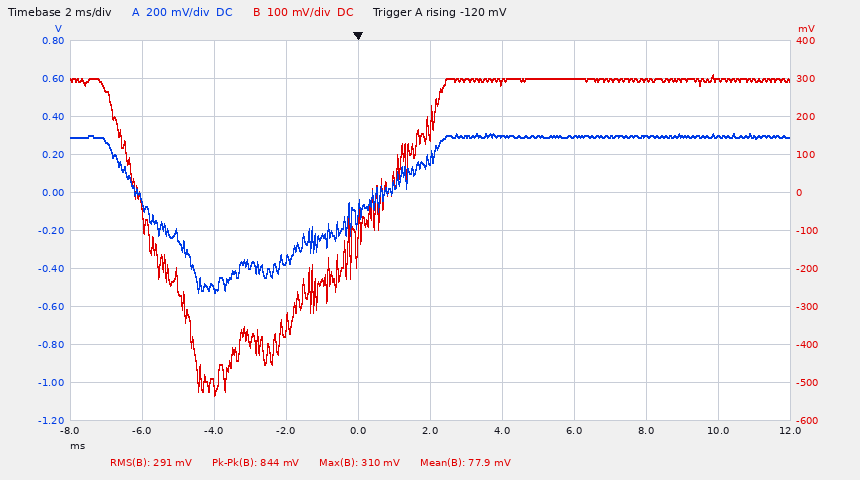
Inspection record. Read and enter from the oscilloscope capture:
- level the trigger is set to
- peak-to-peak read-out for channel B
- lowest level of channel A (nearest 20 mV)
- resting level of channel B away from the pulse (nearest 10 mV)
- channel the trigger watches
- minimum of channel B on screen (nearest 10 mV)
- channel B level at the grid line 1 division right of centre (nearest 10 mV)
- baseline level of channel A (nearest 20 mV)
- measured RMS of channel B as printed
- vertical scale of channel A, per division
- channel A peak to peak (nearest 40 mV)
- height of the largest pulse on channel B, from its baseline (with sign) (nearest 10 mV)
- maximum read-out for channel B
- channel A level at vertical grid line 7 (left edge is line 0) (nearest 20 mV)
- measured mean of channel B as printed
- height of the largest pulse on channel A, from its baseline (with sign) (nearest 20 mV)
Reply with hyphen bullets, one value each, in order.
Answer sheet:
- -120 mV
- 844 mV
- -520 mV
- 300 mV
- channel A
- -530 mV
- 290 mV
- 300 mV
- 291 mV
- 200 mV
- 840 mV
- -830 mV
- 310 mV
- 300 mV
- 77.9 mV
- -820 mV
